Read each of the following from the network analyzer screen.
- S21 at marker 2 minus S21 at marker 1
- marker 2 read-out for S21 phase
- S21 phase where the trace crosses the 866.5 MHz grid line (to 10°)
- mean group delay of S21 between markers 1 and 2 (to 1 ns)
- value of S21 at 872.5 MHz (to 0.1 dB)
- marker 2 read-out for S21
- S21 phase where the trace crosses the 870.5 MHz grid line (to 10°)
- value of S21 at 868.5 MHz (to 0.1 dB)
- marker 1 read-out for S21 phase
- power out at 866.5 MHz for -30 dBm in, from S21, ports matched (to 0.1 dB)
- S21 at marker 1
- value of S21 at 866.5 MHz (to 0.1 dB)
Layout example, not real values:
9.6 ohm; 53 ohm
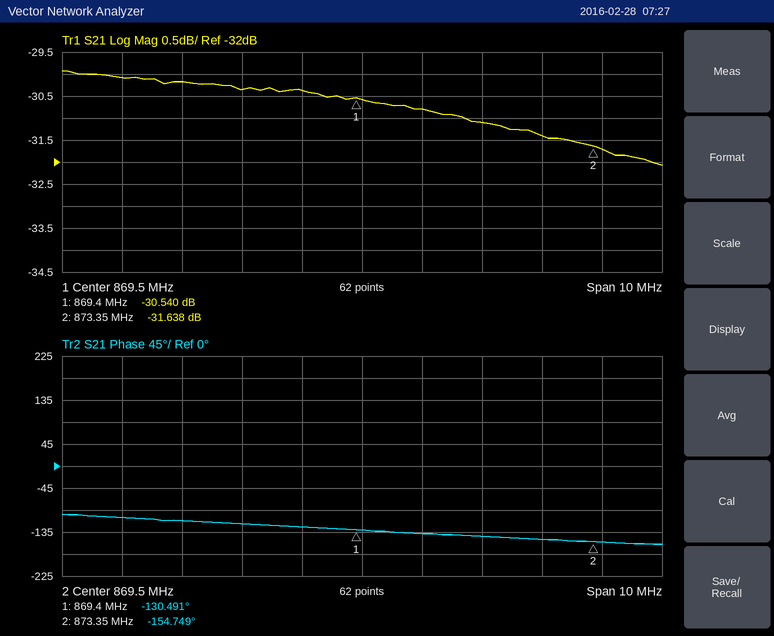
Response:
-1.098 dB; -154.749°; -110°; 17 ns; -31.4 dB; -31.638 dB; -140°; -30.4 dB; -130.491°; -60.2 dBm; -30.540 dB; -30.2 dB
